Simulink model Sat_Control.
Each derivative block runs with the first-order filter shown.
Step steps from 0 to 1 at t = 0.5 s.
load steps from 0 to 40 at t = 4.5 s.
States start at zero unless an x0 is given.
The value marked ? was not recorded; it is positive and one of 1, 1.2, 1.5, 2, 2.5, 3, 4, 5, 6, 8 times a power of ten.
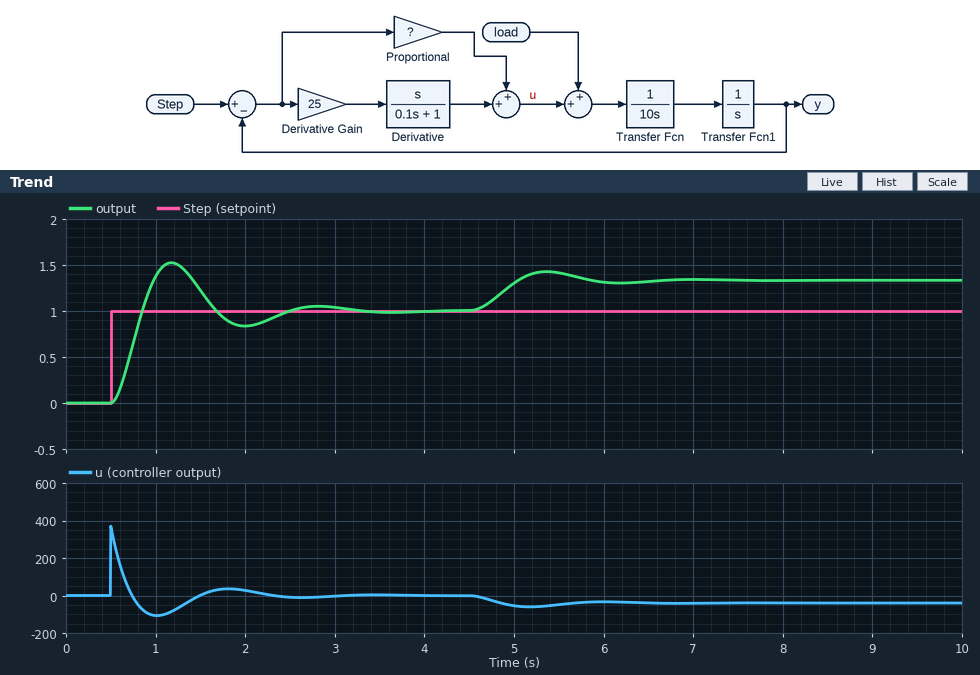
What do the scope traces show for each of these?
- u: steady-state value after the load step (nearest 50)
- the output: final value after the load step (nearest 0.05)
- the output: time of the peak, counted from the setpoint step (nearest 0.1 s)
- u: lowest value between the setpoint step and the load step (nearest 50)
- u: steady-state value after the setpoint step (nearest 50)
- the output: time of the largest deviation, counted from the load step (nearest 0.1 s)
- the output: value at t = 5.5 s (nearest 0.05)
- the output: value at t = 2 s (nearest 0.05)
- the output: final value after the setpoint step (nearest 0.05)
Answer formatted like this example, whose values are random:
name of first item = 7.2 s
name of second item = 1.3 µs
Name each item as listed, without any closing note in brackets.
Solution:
u: steady-state value after the load step = -50
the output: final value after the load step = 1.35
the output: time of the peak, counted from the setpoint step = 0.7 s
u: lowest value between the setpoint step and the load step = -100
u: steady-state value after the setpoint step = 0
the output: time of the largest deviation, counted from the load step = 0.9 s
the output: value at t = 5.5 s = 1.40
the output: value at t = 2 s = 0.85
the output: final value after the setpoint step = 1.00
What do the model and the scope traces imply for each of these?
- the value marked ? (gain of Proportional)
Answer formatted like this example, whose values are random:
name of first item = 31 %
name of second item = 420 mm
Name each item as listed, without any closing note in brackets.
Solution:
the value marked ? = 120
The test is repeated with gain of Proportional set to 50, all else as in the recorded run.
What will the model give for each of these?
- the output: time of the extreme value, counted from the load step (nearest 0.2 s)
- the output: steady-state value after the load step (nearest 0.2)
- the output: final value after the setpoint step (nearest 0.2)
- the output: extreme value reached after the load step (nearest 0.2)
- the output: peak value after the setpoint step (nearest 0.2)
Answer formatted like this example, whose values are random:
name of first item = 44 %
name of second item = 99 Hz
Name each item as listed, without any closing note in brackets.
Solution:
the output: time of the extreme value, counted from the load step = 1.6 s
the output: steady-state value after the load step = 1.8
the output: final value after the setpoint step = 1.0
the output: extreme value reached after the load step = 1.8
the output: peak value after the setpoint step = 1.4
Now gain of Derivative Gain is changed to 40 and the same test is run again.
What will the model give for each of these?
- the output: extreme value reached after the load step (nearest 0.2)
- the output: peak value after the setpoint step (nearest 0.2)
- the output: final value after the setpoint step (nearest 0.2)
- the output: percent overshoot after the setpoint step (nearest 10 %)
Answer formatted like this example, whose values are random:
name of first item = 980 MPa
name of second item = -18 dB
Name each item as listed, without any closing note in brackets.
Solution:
the output: extreme value reached after the load step = 1.4
the output: peak value after the setpoint step = 1.4
the output: final value after the setpoint step = 1.0
the output: percent overshoot after the setpoint step = 40 %
